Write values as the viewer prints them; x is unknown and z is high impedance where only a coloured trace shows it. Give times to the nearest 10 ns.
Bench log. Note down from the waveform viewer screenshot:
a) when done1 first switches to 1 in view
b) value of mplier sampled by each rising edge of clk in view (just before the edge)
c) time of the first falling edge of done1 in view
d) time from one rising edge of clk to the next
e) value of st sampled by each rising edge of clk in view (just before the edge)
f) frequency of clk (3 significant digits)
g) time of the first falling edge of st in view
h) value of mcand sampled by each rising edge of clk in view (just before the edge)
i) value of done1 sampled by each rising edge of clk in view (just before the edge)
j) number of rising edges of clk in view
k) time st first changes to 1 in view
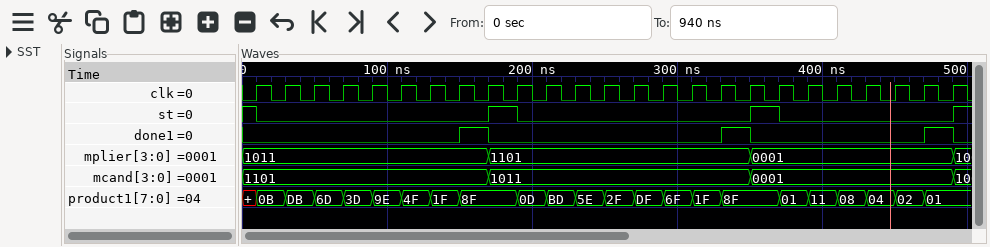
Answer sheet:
150 ns
1011, 1011, 1011, 1011, 1011, 1011, 1011, 1011, 1011, 1101, 1101, 1101, 1101, 1101, 1101, 1101, 1101, 1101, 0001, 0001, 0001, 0001, 0001, 0001, 0001
170 ns
20 ns
1 0 0 0 0 0 0 0 0 1 0 0 0 0 0 0 0 0 1 0 0 0 0 0 0
50.0 MHz
10 ns
1101, 1101, 1101, 1101, 1101, 1101, 1101, 1101, 1101, 1011, 1011, 1011, 1011, 1011, 1011, 1011, 1011, 1011, 0001, 0001, 0001, 0001, 0001, 0001, 0001
0 0 0 0 0 0 0 0 1 0 0 0 0 0 0 0 0 1 0 0 0 0 0 0 1
25
170 ns
